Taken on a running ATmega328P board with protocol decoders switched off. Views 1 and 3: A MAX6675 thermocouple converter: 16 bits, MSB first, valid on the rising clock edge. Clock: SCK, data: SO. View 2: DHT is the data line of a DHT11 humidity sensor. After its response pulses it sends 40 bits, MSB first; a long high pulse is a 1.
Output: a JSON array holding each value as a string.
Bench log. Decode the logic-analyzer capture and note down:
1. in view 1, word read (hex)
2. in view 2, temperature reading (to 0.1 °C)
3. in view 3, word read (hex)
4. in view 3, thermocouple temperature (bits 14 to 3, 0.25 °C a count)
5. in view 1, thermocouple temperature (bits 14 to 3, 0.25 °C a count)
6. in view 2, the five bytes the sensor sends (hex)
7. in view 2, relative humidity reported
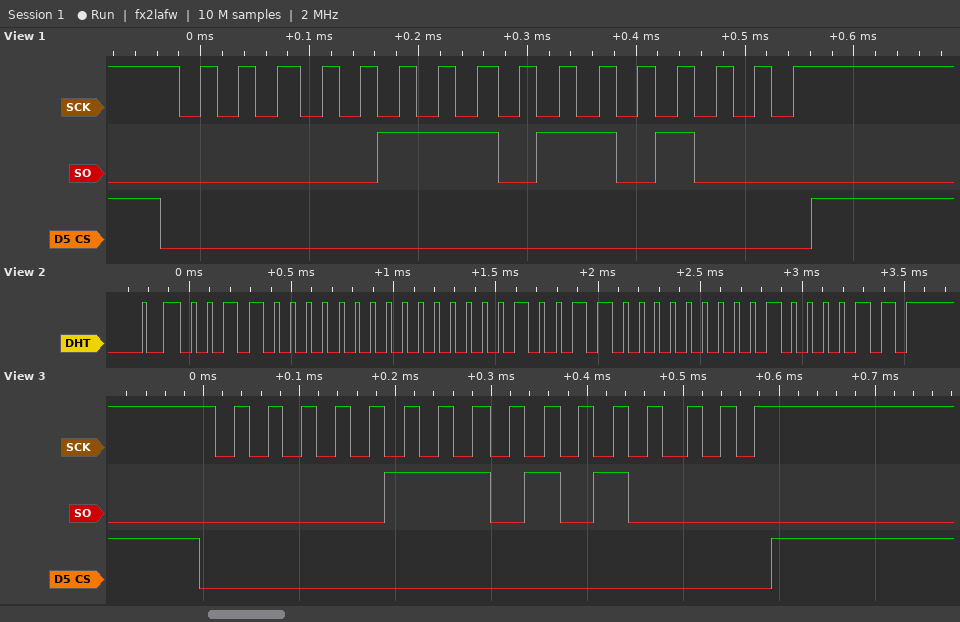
["0x0768", "19.0 °C", "0x0750", "58.50 °C", "59.25 °C", "30 00 13 00 43", "48 %"]
